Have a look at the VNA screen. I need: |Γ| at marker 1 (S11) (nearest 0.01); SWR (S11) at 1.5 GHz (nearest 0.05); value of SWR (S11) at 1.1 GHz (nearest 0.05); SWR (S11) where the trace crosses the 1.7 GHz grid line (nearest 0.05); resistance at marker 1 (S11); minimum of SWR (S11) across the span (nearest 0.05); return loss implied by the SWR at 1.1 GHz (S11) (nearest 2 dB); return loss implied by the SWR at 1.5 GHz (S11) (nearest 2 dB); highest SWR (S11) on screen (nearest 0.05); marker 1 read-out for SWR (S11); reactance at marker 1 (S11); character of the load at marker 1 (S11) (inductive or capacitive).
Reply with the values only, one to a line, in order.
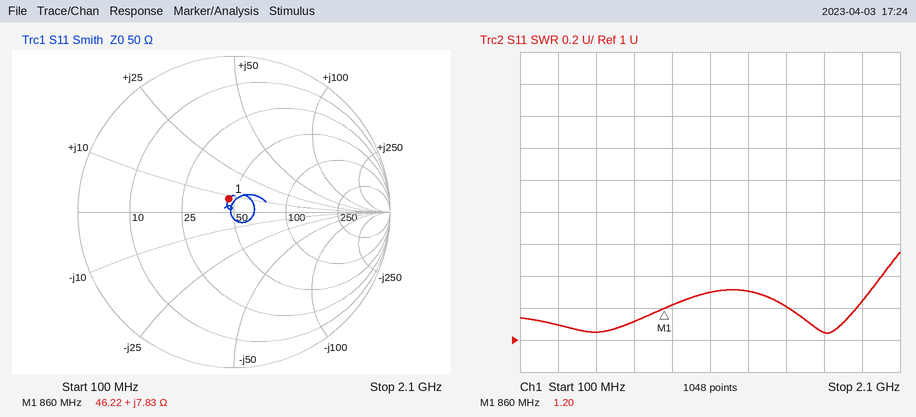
0.09
1.20
1.30
1.05
46.22 Ω
1.05
18 dB
20 dB
1.55
1.20
+7.83 Ω
inductive
